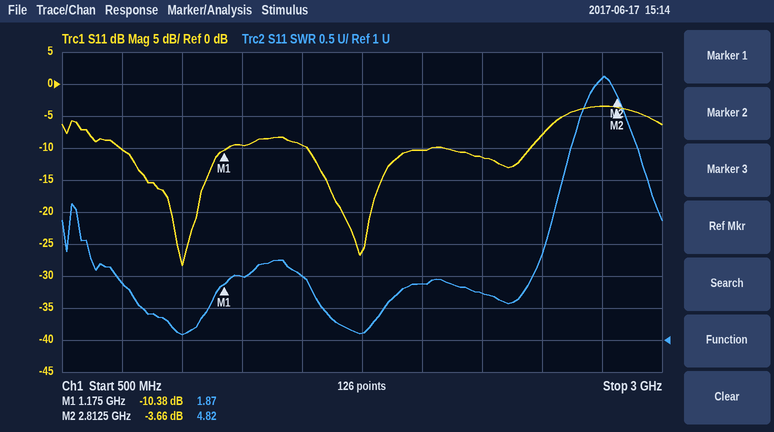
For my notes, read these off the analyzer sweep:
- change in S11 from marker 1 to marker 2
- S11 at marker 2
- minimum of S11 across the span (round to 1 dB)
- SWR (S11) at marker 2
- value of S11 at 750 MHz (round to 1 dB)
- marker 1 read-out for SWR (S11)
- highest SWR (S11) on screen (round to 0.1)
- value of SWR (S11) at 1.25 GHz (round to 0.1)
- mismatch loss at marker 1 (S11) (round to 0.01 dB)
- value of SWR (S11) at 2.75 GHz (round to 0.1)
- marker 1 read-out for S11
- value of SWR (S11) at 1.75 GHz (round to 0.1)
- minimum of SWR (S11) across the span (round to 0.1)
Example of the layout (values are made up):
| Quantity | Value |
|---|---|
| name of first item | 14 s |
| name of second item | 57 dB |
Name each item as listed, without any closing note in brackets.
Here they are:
| Quantity | Value |
|---|---|
| change in S11 from marker 1 to marker 2 | 6.72 dB |
| S11 at marker 2 | -3.66 dB |
| minimum of S11 across the span | -28 dB |
| SWR (S11) at marker 2 | 4.82 |
| value of S11 at 750 MHz | -10 dB |
| marker 1 read-out for SWR | 1.87 |
| highest SWR (S11) on screen | 5.1 |
| value of SWR (S11) at 1.25 GHz | 2.0 |
| mismatch loss at marker 1 (S11) | 0.42 dB |
| value of SWR (S11) at 2.75 GHz | 5.1 |
| marker 1 read-out for S11 | -10.38 dB |
| value of SWR (S11) at 1.75 GHz | 1.1 |
| minimum of SWR (S11) across the span | 1.1 |
